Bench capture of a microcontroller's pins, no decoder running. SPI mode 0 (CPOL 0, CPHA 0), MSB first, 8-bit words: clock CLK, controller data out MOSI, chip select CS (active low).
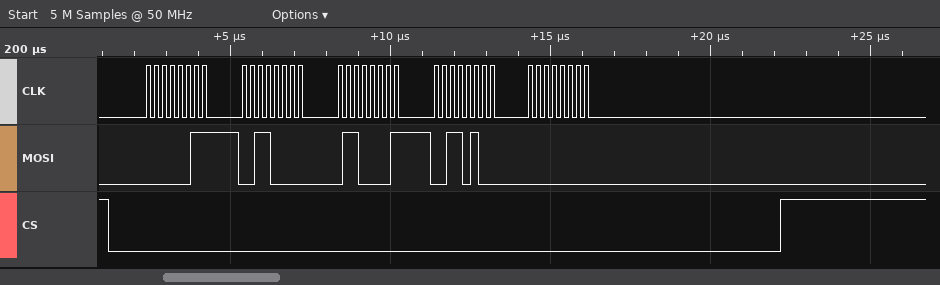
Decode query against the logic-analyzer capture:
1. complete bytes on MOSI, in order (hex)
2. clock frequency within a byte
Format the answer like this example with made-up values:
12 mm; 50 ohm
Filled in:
03 30 61 34 00; 4 MHz
